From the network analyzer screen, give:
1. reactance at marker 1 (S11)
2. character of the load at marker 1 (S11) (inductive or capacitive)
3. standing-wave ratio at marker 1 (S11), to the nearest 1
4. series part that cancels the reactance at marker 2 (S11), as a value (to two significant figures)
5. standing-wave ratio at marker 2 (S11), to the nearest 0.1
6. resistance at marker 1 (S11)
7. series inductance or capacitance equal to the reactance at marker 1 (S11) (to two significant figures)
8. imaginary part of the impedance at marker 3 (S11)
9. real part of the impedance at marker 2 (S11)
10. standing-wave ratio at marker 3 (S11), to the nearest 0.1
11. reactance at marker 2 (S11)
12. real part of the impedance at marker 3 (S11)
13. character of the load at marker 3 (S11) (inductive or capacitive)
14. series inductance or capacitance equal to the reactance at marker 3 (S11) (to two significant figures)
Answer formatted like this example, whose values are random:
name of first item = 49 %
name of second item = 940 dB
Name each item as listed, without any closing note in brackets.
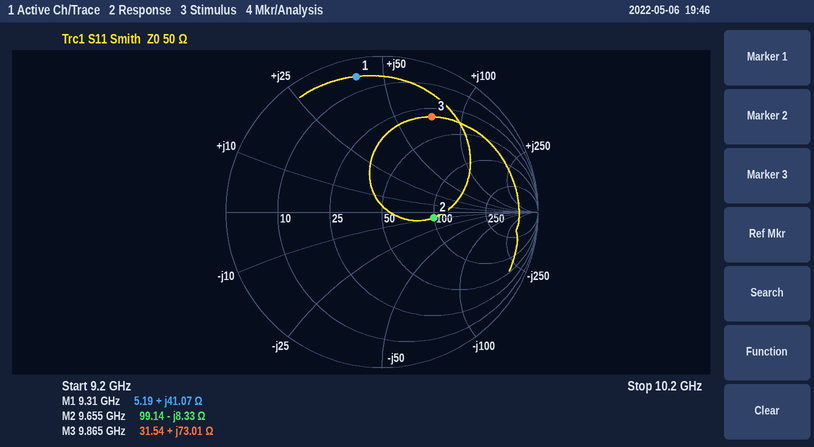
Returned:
reactance at marker 1 = +41.07 Ω
character of the load at marker 1 (S11) = inductive
standing-wave ratio at marker 1 (S11), to the nearest 1 = 16
series part that cancels the reactance at marker 2 (S11), as a value = 140 pH
standing-wave ratio at marker 2 (S11), to the nearest 0.1 = 2.0
resistance at marker 1 = 5.19 Ω
series inductance or capacitance equal to the reactance at marker 1 (S11) = 700 pH
imaginary part of the impedance at marker 3 = +73.01 Ω
real part of the impedance at marker 2 = 99.14 Ω
standing-wave ratio at marker 3 (S11), to the nearest 0.1 = 5.4
reactance at marker 2 = -8.33 Ω
real part of the impedance at marker 3 = 31.54 Ω
character of the load at marker 3 (S11) = inductive
series inductance or capacitance equal to the reactance at marker 3 (S11) = 1.2 nH
